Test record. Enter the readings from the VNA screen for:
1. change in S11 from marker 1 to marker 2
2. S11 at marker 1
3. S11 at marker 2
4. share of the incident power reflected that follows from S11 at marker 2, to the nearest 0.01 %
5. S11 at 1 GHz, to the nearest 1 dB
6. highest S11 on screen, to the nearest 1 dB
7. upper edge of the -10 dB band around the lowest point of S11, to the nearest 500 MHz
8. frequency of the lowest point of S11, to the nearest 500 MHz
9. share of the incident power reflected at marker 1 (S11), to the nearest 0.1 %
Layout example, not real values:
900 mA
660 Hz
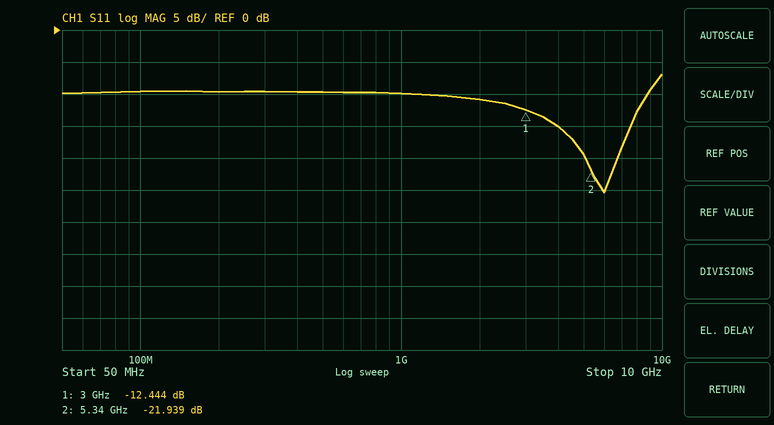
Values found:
-9.495 dB
-12.444 dB
-21.939 dB
0.64 %
-10 dB
-7 dB
9.0 GHz
6.0 GHz
5.7 %
